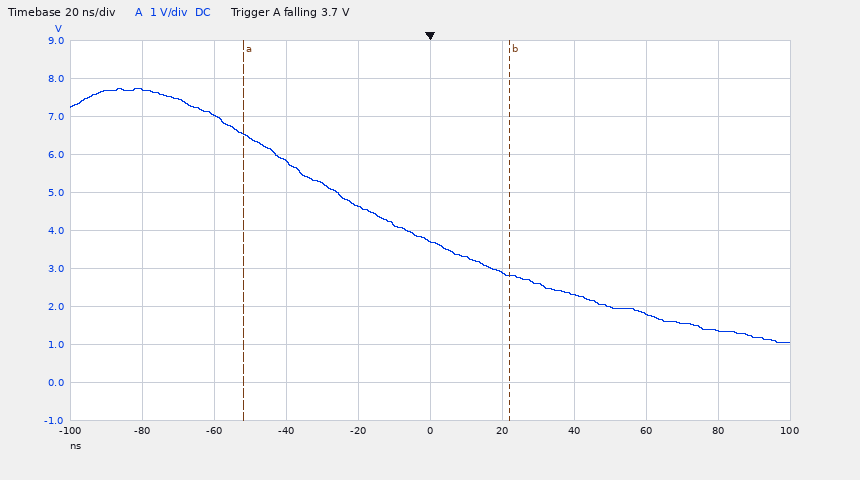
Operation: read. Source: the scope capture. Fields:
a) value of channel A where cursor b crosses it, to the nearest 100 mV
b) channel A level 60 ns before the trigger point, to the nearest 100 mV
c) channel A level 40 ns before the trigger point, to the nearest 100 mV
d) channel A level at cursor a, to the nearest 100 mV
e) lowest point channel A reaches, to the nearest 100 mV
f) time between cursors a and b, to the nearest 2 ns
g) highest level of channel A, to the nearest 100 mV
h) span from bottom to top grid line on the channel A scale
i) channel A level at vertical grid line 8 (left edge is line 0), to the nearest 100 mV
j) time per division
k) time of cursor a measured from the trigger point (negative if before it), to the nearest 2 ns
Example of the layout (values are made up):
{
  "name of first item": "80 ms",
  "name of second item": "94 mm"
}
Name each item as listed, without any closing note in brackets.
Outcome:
{
  "value of channel A where cursor b crosses it, to the nearest 100 mV": "2.8 V",
  "channel A level 60 ns before the trigger point, to the nearest 100 mV": "7.0 V",
  "channel A level 40 ns before the trigger point, to the nearest 100 mV": "5.8 V",
  "channel A level at cursor a, to the nearest 100 mV": "6.5 V",
  "lowest point channel A reaches, to the nearest 100 mV": "1.1 V",
  "time between cursors a and b, to the nearest 2 ns": "74 ns",
  "highest level of channel A, to the nearest 100 mV": "7.7 V",
  "span from bottom to top grid line on the channel A scale": "10 V",
  "channel A level at vertical grid line 8 (left edge is line 0), to the nearest 100 mV": "1.8 V",
  "time per division": "20 ns",
  "time of cursor a measured from the trigger point (negative if before it), to the nearest 2 ns": "-52 ns"
}
